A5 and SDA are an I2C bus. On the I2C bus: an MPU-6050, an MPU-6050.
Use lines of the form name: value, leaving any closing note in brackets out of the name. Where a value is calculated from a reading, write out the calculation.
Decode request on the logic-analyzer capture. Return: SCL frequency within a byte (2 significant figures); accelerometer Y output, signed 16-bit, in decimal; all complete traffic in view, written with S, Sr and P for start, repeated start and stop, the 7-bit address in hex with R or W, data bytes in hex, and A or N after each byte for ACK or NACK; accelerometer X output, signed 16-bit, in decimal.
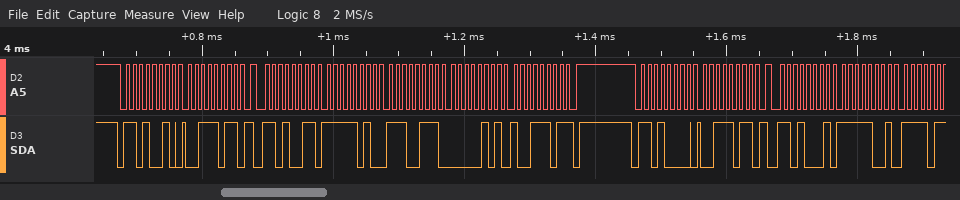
SCL frequency within a byte: 100 kHz
accelerometer Y output, signed 16-bit, in decimal: 0x059D = 1437
all complete traffic in view, written with S, Sr and P for start, repeated start and stop, the 7-bit address in hex with R or W, data bytes in hex, and A or N after each byte for ACK or NACK: S 69W A 3B A Sr 69R A FA A E7 A 05 A 9D N P S 68W A 3B A Sr 68R A F9 A
accelerometer X output, signed 16-bit, in decimal: 0xFAE7 = -1305
